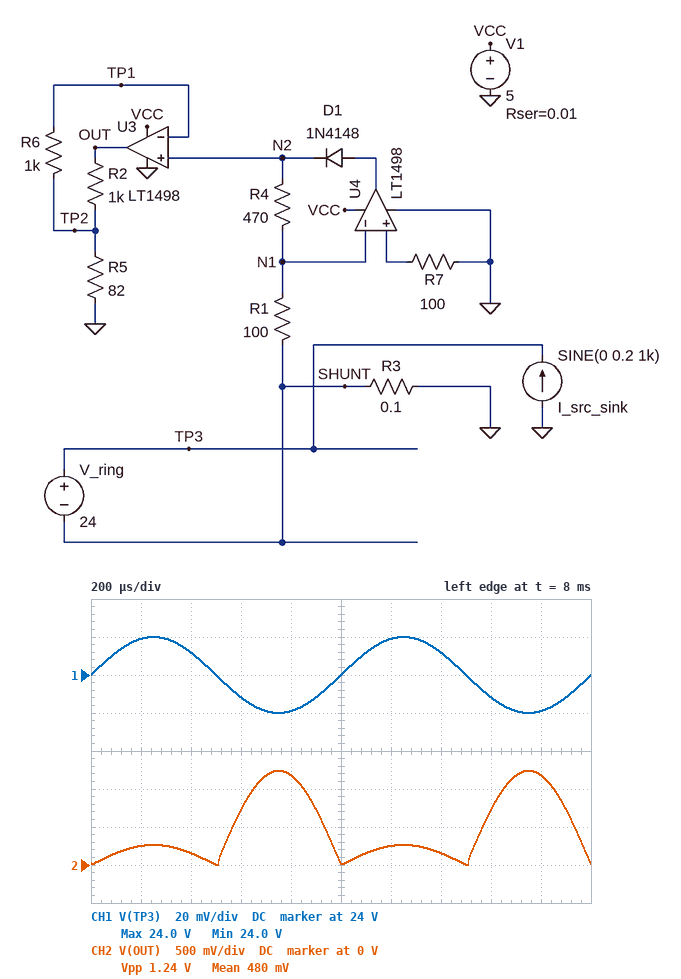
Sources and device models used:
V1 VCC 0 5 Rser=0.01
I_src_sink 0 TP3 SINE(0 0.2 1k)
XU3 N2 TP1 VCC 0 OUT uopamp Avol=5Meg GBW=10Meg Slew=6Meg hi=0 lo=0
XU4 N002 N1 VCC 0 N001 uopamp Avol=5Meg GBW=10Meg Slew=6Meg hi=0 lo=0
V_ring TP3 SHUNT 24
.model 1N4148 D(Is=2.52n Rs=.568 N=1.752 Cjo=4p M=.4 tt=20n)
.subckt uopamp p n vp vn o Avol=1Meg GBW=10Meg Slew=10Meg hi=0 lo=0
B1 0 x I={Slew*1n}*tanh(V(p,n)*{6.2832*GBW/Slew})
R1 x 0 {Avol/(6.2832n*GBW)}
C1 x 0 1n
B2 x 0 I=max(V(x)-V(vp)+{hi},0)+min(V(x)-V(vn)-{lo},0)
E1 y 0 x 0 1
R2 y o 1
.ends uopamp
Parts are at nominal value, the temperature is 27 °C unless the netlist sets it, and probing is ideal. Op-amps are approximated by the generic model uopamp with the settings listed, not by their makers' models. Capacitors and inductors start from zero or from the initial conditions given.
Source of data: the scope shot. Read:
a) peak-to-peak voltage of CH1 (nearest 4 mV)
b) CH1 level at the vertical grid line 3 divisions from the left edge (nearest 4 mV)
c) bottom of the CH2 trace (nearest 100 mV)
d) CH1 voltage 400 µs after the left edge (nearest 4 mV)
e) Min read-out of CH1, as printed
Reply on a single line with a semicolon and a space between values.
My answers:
40 mV; 23.988 V; 0 V; 24.012 V; 24.0 V
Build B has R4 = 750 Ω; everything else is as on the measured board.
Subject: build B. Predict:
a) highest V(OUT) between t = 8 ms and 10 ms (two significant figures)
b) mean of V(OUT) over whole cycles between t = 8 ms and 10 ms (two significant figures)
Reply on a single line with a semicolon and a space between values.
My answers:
2.0 V; 710 mV
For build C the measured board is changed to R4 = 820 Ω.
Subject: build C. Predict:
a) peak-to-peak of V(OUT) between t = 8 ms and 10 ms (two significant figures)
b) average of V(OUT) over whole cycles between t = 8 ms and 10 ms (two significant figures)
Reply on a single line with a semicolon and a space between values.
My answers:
2.2 V; 770 mV
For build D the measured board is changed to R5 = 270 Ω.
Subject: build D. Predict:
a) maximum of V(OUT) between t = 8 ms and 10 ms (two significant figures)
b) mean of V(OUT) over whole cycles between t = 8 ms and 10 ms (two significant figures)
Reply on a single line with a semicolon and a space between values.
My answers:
440 mV; 170 mV
